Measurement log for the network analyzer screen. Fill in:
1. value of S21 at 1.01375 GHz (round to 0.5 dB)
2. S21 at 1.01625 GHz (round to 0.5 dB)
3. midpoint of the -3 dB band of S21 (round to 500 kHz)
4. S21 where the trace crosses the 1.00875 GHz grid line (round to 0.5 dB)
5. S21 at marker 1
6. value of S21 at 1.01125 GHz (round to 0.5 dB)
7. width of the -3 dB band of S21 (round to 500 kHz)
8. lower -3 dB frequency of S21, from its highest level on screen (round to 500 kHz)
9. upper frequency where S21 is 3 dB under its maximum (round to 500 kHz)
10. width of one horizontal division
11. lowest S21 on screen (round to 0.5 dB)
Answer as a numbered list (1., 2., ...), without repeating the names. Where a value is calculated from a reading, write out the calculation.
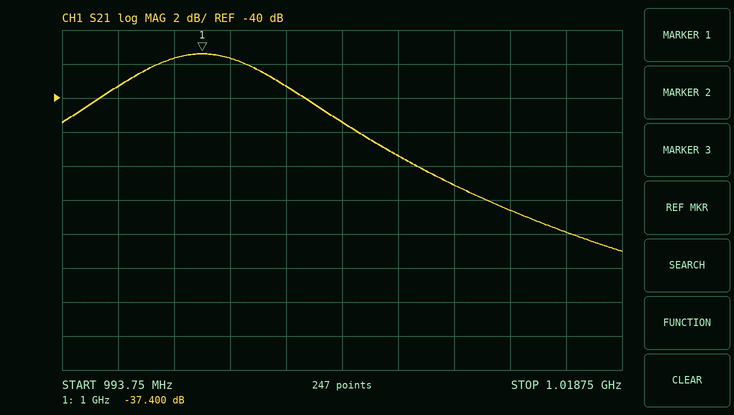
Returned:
1. -46.5 dB
2. -48.0 dB
3. 1.0000 GHz
4. -43.5 dB
5. -37.400 dB
6. -45.0 dB
7. 1.0050 GHz − 995.0 MHz = 10.0 MHz
8. 995.0 MHz
9. 1.0050 GHz
10. 2.5 MHz
11. -49.0 dB
